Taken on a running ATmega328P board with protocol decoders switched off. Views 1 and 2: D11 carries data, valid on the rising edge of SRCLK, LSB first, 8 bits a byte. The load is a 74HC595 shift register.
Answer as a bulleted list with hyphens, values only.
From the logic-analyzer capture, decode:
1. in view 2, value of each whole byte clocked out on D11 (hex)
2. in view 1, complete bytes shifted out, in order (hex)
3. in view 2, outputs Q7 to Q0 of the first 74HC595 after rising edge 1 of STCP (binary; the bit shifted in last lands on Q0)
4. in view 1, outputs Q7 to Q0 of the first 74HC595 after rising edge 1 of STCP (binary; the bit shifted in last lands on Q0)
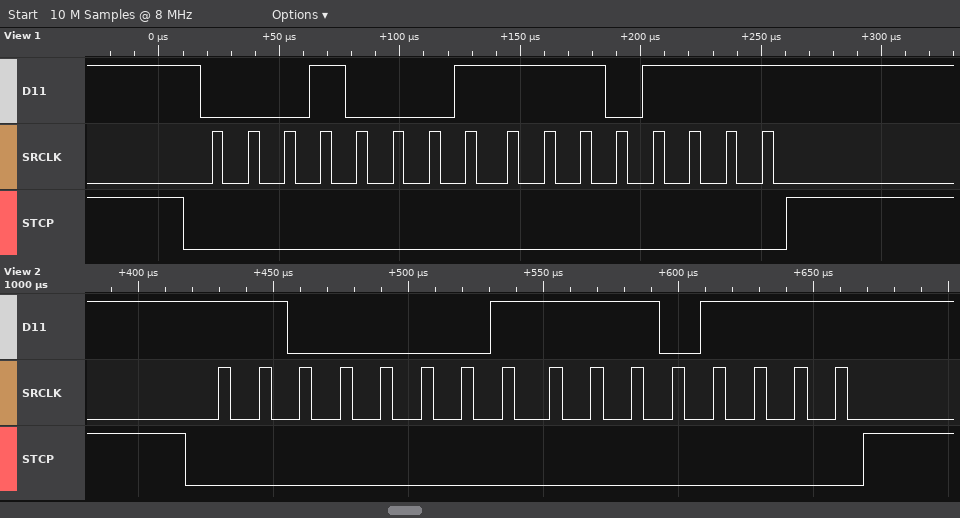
- 83 F7
- 0x88 0xF7
- 11101111
- 11101111
